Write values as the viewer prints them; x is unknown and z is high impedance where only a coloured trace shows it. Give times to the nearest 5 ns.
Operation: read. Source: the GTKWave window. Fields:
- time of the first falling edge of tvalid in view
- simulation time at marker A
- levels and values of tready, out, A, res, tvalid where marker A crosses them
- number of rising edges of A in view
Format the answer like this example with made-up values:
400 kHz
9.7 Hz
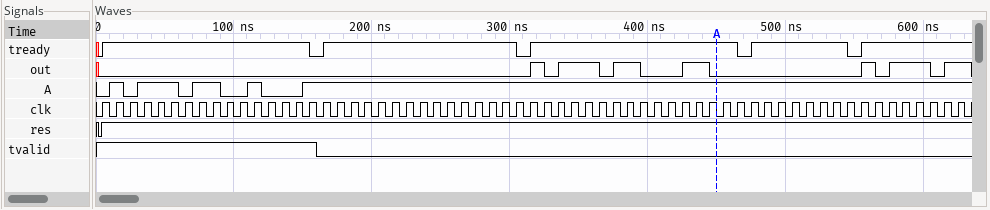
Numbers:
160 ns
450 ns
tready=1, out=0, A=1, res=1, tvalid=0
5
